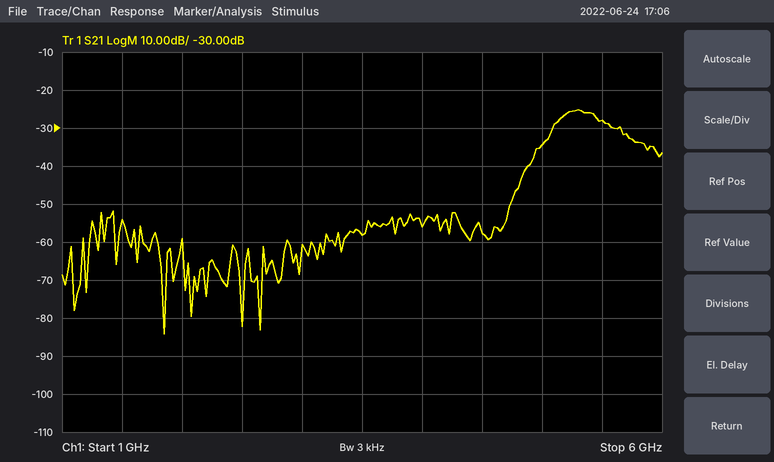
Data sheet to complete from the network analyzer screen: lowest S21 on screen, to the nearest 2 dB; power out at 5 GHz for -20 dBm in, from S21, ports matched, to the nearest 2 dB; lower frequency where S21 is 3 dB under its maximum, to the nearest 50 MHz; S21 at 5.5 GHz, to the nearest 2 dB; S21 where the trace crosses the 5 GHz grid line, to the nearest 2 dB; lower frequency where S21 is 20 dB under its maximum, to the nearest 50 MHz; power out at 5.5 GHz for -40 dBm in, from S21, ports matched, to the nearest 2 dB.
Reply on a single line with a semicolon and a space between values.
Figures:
-84 dB; -54 dBm; 5.15 GHz; -28 dB; -34 dB; 4.80 GHz; -68 dBm
